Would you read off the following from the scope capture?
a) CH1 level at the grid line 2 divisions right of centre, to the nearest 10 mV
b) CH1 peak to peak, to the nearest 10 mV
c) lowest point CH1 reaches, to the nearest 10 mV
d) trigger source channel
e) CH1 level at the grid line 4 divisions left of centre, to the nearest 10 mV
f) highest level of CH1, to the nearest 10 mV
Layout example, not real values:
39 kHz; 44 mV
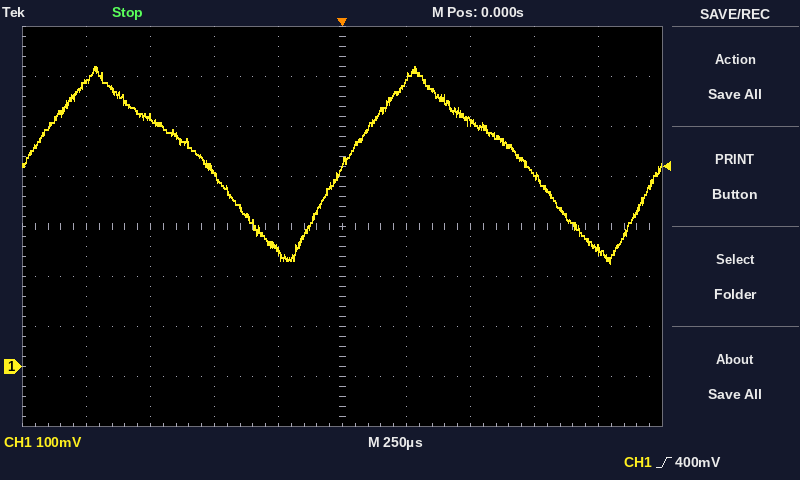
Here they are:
490 mV; 390 mV; 210 mV; CH1; 570 mV; 600 mV
